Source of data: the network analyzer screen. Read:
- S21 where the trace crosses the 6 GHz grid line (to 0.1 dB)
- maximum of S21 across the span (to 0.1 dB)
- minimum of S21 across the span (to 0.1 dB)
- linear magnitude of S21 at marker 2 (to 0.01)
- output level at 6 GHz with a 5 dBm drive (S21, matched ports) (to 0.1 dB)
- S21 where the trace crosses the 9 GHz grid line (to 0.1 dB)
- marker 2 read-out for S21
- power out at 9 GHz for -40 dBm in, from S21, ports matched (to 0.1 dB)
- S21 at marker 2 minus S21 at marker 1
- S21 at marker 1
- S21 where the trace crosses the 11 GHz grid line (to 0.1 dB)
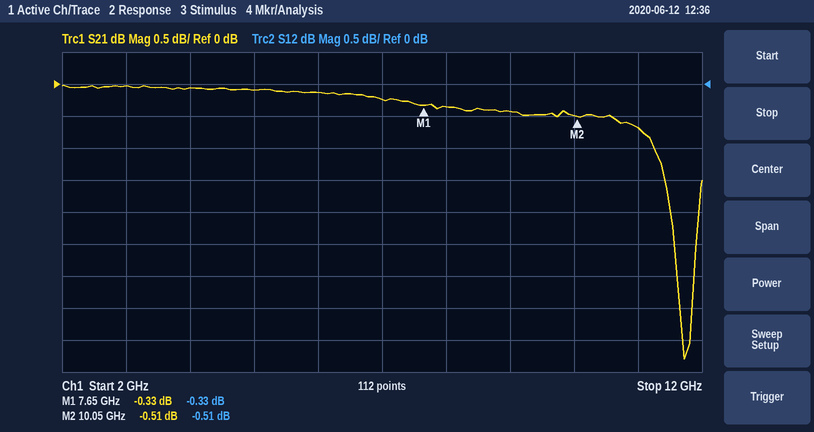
-0.1 dB
0.0 dB
-4.3 dB
0.94
4.9 dBm
-0.4 dB
-0.51 dB
-40.4 dBm
-0.18 dB
-0.33 dB
-0.7 dB
